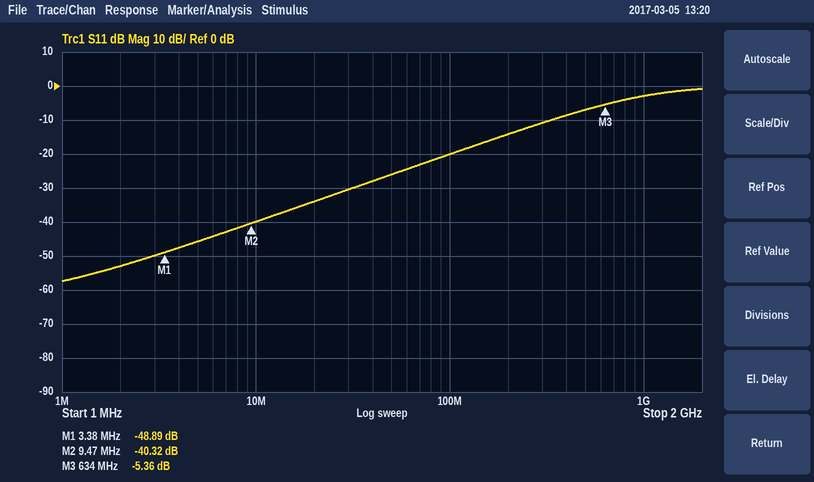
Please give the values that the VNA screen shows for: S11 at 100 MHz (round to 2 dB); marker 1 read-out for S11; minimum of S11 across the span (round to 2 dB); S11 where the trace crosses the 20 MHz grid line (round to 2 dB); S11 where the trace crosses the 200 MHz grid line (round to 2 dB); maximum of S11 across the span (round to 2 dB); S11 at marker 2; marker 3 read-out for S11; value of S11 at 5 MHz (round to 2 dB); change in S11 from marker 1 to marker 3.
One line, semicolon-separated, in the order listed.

-20 dB; -48.89 dB; -58 dB; -34 dB; -14 dB; 0 dB; -40.32 dB; -5.36 dB; -46 dB; 43.53 dB
